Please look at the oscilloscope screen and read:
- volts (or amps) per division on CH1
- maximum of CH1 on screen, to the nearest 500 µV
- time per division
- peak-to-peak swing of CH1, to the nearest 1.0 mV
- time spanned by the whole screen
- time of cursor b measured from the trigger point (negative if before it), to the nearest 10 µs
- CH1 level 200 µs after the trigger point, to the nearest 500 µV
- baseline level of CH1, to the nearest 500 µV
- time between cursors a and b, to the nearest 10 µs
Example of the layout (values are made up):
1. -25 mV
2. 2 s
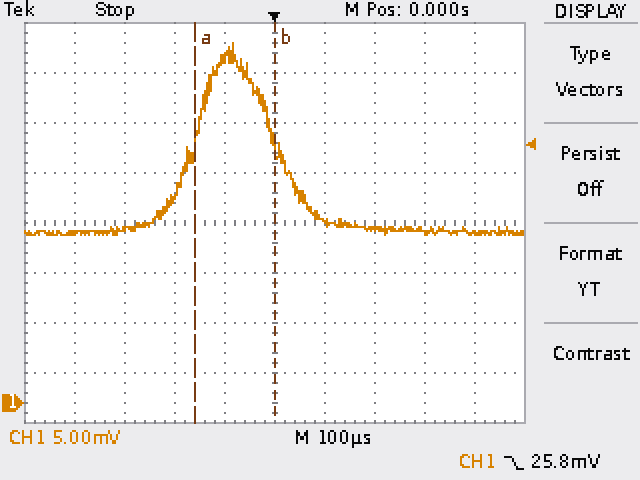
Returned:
1. 5 mV
2. 36.0 mV
3. 100 µs
4. 19.0 mV
5. 1 ms
6. 0 µs
7. 17.5 mV
8. 17.0 mV
9. 160 µs
